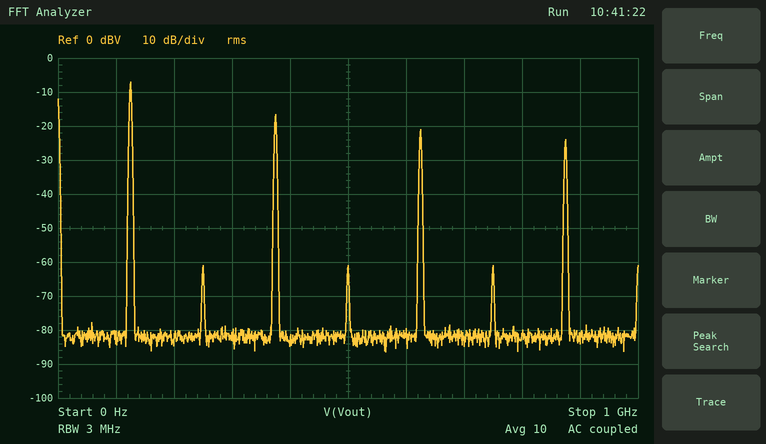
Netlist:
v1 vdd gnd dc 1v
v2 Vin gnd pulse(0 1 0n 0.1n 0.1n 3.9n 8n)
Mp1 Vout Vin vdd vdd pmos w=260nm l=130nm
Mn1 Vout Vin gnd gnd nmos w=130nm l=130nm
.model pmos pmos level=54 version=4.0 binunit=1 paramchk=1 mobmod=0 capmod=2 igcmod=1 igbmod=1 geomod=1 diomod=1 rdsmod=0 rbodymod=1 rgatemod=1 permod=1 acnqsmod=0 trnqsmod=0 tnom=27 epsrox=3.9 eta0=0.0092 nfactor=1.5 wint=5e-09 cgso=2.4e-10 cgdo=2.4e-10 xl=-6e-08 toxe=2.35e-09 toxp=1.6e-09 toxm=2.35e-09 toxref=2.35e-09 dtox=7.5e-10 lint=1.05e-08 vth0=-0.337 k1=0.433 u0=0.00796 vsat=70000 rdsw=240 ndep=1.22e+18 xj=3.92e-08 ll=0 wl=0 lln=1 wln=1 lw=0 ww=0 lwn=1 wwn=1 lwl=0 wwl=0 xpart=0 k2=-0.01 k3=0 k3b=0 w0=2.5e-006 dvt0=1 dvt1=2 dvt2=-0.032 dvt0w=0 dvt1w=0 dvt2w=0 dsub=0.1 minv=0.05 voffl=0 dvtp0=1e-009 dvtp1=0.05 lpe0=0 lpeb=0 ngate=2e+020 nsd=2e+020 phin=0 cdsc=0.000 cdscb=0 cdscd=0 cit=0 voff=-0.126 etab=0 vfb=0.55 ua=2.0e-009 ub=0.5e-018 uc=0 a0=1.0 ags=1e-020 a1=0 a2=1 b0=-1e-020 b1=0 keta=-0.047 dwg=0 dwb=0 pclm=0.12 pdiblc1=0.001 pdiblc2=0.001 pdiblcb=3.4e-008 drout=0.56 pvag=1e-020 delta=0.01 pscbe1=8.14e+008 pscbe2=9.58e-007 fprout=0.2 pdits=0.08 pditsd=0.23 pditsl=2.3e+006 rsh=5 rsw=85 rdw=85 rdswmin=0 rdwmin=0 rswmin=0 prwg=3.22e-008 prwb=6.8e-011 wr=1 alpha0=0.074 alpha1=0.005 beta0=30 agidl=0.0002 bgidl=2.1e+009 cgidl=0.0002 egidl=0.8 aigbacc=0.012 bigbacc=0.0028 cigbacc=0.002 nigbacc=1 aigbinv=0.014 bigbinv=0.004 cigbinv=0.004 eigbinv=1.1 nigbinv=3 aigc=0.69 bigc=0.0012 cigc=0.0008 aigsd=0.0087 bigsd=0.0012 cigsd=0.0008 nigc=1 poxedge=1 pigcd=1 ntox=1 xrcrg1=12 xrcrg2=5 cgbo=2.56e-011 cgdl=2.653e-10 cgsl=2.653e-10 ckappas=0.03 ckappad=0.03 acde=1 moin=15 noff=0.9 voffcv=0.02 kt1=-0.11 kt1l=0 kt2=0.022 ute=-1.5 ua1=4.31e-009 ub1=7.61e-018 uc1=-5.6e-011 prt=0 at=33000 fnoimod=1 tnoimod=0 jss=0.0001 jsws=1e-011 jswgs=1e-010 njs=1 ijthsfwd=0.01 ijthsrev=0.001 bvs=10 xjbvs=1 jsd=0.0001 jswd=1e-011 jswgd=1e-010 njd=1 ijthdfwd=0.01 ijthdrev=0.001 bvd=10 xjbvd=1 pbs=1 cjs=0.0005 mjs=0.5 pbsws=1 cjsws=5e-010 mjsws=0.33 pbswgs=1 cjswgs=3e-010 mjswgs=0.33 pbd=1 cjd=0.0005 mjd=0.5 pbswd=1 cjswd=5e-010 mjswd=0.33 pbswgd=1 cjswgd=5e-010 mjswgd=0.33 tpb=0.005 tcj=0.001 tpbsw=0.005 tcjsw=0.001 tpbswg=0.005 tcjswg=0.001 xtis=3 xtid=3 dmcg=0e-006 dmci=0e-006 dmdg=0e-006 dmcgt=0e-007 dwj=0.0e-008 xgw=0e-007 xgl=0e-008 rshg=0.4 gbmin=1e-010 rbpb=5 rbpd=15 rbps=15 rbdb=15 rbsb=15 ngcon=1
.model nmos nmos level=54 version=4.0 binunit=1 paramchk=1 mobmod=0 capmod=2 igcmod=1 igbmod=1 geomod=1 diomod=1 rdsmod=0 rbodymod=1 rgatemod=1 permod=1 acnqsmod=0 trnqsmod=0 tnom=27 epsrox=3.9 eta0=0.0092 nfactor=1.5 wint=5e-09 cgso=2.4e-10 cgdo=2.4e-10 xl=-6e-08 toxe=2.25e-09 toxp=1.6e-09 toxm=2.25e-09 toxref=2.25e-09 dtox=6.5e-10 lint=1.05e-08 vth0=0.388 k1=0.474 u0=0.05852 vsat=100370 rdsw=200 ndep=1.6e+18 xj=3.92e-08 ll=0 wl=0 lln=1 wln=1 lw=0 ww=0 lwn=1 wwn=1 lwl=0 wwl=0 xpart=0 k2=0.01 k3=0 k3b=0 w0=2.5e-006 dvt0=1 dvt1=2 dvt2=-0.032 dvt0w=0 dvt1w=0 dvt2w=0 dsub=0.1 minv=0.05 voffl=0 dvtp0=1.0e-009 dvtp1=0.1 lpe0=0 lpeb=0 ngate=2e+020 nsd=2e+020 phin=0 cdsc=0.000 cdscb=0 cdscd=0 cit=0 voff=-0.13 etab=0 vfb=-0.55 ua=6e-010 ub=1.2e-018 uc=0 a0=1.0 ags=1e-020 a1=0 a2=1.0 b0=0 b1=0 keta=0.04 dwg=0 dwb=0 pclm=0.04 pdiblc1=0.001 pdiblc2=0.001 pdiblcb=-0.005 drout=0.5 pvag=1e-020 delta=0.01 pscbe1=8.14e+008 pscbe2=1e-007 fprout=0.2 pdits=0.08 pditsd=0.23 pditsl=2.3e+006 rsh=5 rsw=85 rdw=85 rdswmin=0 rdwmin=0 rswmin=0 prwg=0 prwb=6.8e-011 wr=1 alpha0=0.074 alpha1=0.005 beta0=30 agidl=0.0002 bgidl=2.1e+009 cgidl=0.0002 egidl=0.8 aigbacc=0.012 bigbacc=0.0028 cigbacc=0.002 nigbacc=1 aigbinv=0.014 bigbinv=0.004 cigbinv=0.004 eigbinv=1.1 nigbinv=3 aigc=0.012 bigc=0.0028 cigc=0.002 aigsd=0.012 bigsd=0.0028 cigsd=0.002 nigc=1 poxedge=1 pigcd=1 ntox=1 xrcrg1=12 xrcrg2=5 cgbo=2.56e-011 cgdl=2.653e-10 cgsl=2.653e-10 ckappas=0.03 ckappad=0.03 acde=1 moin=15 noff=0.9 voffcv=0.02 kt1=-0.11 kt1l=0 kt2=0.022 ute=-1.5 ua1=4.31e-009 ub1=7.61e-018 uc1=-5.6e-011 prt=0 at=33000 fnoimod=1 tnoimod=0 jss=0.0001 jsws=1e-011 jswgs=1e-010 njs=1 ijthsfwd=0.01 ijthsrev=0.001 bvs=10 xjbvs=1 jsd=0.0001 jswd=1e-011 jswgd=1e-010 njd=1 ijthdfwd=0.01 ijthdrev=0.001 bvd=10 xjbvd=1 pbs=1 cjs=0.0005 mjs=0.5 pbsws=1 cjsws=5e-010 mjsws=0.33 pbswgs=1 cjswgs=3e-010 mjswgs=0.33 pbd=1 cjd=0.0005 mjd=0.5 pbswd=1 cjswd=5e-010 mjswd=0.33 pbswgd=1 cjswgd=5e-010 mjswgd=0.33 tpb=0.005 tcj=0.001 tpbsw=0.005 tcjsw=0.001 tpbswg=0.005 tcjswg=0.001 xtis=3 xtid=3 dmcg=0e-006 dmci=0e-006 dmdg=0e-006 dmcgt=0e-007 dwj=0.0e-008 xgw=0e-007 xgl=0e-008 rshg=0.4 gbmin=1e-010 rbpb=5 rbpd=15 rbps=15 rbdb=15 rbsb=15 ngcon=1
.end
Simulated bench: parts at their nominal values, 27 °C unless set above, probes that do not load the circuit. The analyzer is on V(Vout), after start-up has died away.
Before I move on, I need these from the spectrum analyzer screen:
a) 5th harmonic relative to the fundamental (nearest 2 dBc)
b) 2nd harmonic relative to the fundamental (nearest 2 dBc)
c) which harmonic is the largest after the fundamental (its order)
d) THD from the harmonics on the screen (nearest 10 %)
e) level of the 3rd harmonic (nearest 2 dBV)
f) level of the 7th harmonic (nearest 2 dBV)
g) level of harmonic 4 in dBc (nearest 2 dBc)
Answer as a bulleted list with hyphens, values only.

- -14 dBc
- -54 dBc
- 3
- 40 %
- -16 dBV
- -24 dBV
- -54 dBc
